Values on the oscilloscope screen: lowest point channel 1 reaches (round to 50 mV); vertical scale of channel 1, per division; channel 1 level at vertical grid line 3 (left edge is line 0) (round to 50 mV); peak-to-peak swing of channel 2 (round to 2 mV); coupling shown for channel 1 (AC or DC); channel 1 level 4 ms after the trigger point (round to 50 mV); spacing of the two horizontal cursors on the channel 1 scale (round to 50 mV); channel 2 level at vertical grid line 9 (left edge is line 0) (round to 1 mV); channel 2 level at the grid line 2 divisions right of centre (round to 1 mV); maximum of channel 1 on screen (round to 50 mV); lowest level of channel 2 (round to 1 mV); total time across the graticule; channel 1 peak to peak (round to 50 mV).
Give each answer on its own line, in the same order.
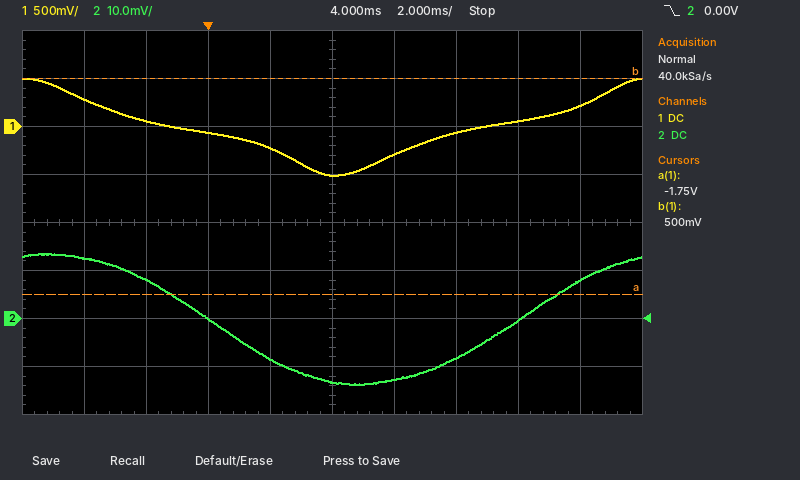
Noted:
-500 mV
500 mV
-50 mV
28 mV
DC
-500 mV
2.25 V
8 mV
-8 mV
500 mV
-14 mV
20 ms
1.00 V
